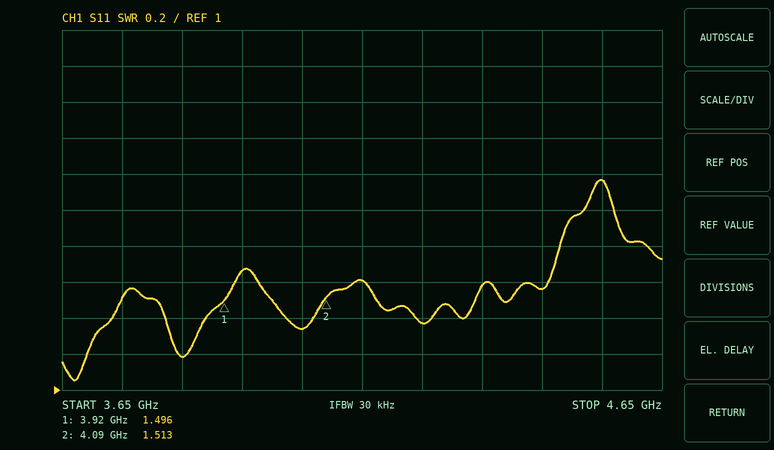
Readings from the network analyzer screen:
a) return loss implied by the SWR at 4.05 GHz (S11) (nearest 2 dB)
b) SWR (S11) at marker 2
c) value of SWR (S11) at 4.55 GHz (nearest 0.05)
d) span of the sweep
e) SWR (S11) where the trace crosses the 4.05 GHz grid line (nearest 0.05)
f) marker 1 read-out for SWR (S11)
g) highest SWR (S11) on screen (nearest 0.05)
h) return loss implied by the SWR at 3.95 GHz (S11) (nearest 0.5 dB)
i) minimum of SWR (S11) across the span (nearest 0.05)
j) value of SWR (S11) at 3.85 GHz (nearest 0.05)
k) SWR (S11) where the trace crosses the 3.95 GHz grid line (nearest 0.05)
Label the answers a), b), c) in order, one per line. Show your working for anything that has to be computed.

a) −20 log10((1.35 − 1)/(1.35 + 1)) ≈ 16 dB
b) 1.513
c) 2.15
d) 1 GHz
e) 1.35
f) 1.496
g) 2.15
h) −20 log10((1.65 − 1)/(1.65 + 1)) ≈ 12.2 dB, so 12.0 dB to the nearest 0.5 dB
i) 1.05
j) 1.20
k) 1.65
